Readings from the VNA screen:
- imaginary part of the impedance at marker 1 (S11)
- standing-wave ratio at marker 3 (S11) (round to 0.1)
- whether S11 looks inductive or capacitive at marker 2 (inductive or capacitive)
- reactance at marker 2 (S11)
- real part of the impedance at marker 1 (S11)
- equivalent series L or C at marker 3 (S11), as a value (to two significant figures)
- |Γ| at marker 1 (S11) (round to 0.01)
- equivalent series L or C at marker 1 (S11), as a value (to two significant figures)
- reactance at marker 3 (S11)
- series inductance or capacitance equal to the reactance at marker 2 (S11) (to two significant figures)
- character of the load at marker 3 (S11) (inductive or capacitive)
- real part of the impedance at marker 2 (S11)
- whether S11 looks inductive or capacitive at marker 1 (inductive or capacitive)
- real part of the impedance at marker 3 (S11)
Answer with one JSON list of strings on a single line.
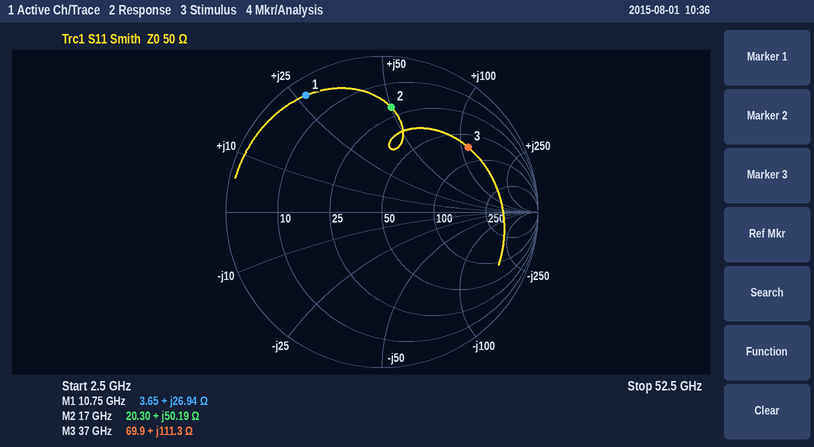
["+26.94 Ω", "5.5", "inductive", "+50.19 Ω", "3.65 Ω", "480 pH", "0.89", "400 pH", "+111.3 Ω", "470 pH", "inductive", "20.30 Ω", "inductive", "69.9 Ω"]
